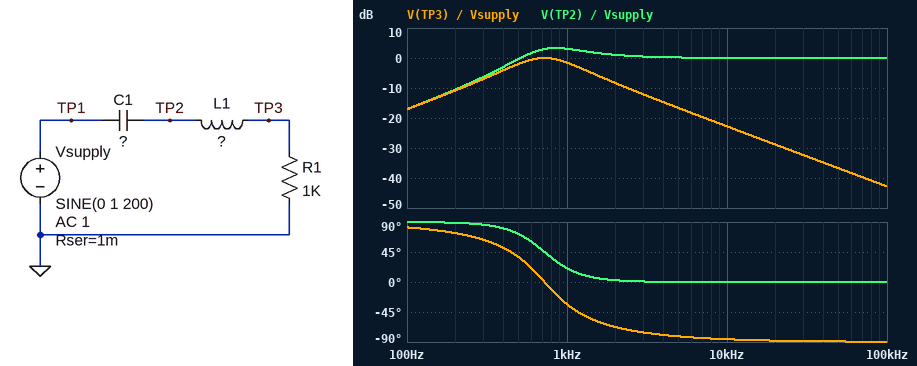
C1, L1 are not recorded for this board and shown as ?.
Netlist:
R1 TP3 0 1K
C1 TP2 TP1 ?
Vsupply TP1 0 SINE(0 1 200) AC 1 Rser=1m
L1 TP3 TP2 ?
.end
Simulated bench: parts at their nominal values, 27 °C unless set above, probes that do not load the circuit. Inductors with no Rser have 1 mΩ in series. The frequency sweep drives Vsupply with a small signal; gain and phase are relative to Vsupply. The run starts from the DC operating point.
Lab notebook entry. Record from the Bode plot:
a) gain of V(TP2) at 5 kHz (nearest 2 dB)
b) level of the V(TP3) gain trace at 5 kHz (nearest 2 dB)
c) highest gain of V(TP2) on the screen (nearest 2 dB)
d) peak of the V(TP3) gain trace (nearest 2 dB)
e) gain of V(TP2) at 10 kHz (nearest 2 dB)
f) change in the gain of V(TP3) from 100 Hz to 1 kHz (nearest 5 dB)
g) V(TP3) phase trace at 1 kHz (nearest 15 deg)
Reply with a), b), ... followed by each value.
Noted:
a) 0 dB
b) -16 dB
c) 4 dB
d) 0 dB
e) 0 dB
f) 15 dB
g) -30 deg
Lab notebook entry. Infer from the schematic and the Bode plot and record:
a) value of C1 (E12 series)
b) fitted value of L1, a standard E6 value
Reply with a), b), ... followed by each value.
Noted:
a) 220 nF
b) 220 mH
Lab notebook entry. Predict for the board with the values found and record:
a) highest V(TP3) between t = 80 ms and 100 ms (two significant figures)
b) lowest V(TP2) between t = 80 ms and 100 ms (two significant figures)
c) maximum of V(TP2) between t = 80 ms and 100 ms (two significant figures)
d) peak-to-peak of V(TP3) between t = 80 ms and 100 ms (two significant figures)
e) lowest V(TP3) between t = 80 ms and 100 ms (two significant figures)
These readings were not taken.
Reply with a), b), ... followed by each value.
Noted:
a) 290 mV
b) -300 mV
c) 300 mV
d) 570 mV
e) -290 mV
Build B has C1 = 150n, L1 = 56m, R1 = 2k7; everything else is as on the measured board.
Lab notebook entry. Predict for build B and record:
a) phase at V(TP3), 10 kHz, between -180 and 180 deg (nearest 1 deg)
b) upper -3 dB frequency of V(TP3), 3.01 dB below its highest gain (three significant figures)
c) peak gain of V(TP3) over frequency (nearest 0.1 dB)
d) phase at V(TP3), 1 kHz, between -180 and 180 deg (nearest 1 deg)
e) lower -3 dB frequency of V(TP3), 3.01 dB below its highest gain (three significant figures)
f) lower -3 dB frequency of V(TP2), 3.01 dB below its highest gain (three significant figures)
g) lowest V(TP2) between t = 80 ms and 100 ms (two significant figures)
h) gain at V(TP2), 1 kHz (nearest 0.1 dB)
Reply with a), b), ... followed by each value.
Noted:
a) -52 deg
b) 8.05 kHz
c) 0 dB
d) 15 deg
e) 375 Hz
f) 402 Hz
g) -460 mV
h) -0.2 dB
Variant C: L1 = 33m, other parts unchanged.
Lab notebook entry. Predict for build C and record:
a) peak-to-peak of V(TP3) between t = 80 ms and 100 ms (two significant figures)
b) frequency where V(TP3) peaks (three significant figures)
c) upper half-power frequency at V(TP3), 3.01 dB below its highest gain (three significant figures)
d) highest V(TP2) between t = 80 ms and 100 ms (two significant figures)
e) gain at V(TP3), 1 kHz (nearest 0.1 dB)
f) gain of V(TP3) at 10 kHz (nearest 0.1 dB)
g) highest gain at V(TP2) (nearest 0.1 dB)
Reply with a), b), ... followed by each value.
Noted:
a) 540 mV
b) 1.87 kHz
c) 5.46 kHz
d) 270 mV
e) -1.0 dB
f) -7.0 dB
g) 0.8 dB
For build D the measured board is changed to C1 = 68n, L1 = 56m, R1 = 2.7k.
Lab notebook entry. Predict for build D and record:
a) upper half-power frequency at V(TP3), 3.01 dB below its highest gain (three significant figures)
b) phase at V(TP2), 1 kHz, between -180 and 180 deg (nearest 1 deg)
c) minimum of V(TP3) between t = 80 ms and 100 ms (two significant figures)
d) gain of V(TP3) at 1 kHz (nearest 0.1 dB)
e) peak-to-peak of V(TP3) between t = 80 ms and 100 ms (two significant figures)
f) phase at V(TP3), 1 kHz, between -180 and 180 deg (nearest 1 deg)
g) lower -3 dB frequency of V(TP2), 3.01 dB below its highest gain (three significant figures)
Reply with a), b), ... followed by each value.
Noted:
a) 8.46 kHz
b) 44 deg
c) -230 mV
d) -1.9 dB
e) 450 mV
f) 36 deg
g) 888 Hz
